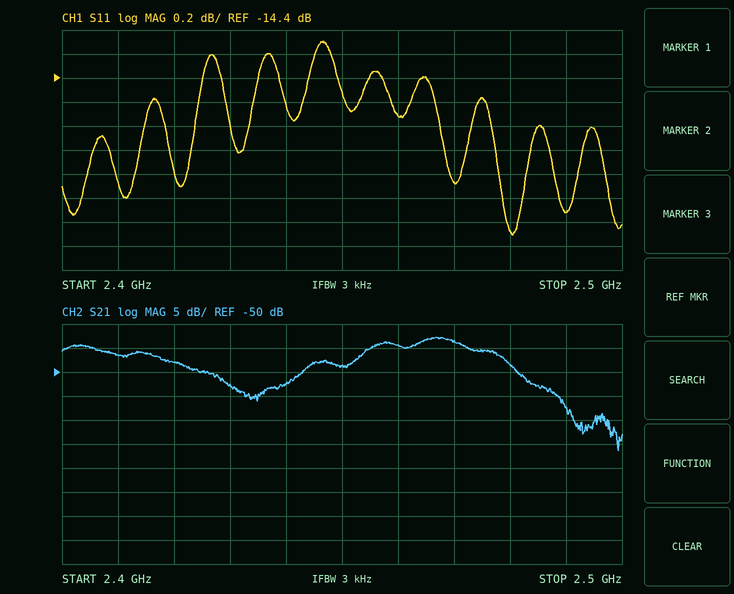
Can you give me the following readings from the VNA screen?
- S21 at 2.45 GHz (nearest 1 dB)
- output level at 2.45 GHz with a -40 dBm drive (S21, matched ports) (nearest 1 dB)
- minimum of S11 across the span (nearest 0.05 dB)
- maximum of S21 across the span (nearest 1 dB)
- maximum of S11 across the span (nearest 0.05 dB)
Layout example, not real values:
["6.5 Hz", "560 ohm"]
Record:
["-49 dB", "-89 dBm", "-15.70 dB", "-43 dB", "-14.10 dB"]
